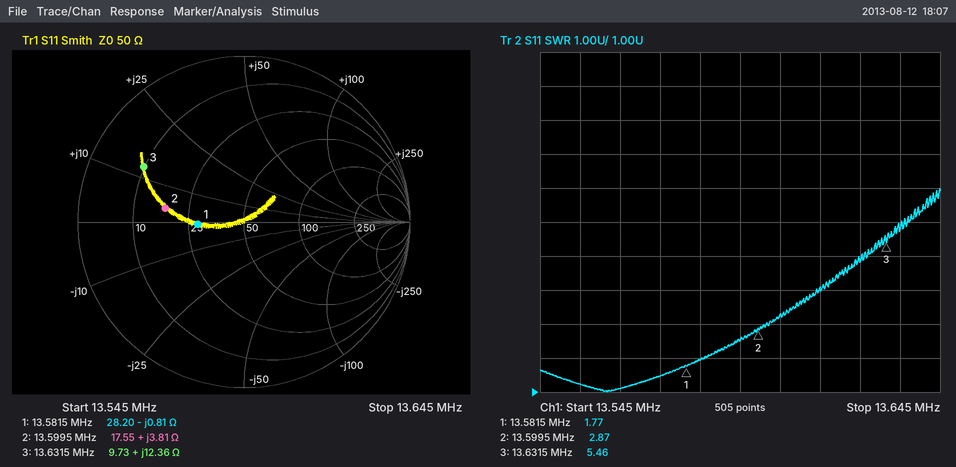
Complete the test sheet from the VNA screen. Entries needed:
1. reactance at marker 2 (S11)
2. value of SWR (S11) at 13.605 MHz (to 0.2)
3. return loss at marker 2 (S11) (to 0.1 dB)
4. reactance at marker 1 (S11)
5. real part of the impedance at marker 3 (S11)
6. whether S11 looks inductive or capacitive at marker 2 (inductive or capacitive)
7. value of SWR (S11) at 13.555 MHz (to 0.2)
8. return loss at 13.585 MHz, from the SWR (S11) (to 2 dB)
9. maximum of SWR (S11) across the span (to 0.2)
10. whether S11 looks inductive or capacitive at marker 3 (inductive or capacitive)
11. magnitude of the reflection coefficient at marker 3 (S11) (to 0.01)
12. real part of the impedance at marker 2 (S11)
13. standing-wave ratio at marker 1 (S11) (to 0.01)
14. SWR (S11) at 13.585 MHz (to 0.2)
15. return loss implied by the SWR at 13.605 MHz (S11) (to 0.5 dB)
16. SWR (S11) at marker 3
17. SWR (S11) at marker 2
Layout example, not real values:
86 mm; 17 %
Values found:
+3.81 Ω; 3.2; 6.3 dB; -0.81 Ω; 9.73 Ω; inductive; 1.2; 10 dB; 7.0; inductive; 0.69; 17.55 Ω; 1.77; 2.0; 5.5 dB; 5.46; 2.87
